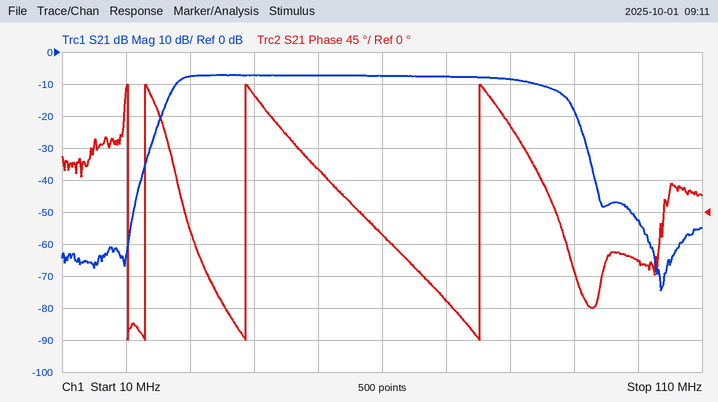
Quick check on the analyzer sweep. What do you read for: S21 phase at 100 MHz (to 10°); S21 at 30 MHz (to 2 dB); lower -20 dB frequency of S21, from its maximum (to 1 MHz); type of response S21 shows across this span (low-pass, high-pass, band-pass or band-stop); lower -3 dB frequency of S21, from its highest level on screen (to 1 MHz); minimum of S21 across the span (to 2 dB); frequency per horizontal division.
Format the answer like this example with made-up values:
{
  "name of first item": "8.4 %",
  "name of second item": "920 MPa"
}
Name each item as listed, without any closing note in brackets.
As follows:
{
  "S21 phase at 100 MHz": "-70°",
  "S21 at 30 MHz": "-8 dB",
  "lower -20 dB frequency of S21, from its maximum": "24 MHz",
  "type of response S21 shows across this span": "band-pass",
  "lower -3 dB frequency of S21, from its highest level on screen": "28 MHz",
  "minimum of S21 across the span": "-74 dB",
  "frequency per horizontal division": "10 MHz"
}
